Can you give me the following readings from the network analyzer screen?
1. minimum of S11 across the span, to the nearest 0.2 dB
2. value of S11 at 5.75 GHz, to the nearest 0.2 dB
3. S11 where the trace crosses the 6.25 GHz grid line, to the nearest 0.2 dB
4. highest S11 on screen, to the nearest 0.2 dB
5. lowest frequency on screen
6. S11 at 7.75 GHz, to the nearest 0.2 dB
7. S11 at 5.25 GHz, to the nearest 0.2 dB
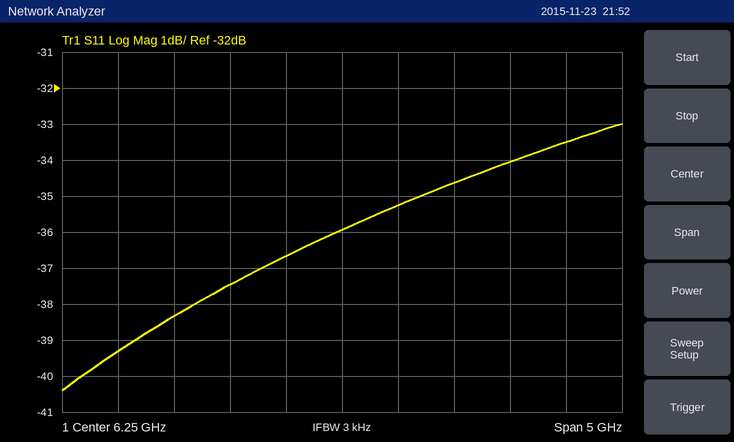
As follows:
-40.4 dB
-36.6 dB
-36.0 dB
-33.0 dB
3.75 GHz
-34.0 dB
-37.4 dB
